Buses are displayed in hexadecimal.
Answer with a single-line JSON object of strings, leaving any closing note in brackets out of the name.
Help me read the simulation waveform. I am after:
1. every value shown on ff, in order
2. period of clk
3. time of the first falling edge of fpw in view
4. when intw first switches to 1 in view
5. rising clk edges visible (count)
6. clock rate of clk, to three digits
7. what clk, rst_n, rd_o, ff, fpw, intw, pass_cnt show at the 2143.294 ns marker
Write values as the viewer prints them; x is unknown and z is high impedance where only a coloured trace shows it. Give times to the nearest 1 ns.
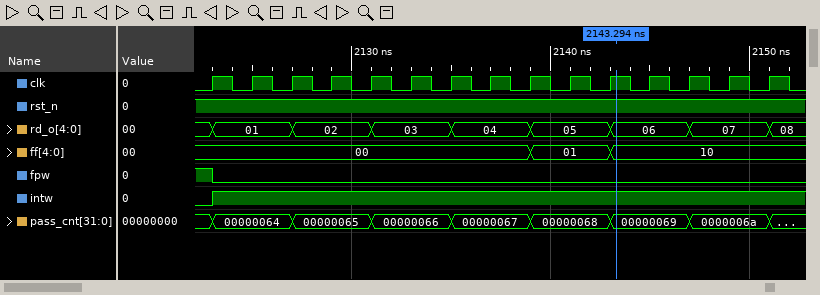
{"every value shown on ff, in order": "00, 01, 10", "period of clk": "2 ns", "time of the first falling edge of fpw in view": "2123 ns", "when intw first switches to 1 in view": "2123 ns", "rising clk edges visible": "15", "clock rate of clk, to three digits": "500 MHz", "what clk, rst_n, rd_o, ff, fpw, intw, pass_cnt show at the 2143.294 ns marker": "clk=1, rst_n=1, rd_o=06, ff=10, fpw=0, intw=1, pass_cnt=00000069"}
